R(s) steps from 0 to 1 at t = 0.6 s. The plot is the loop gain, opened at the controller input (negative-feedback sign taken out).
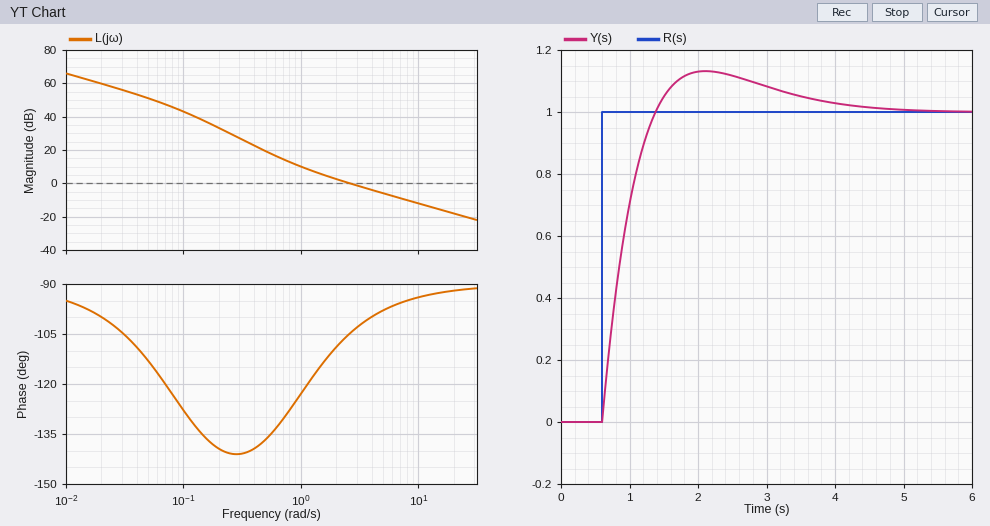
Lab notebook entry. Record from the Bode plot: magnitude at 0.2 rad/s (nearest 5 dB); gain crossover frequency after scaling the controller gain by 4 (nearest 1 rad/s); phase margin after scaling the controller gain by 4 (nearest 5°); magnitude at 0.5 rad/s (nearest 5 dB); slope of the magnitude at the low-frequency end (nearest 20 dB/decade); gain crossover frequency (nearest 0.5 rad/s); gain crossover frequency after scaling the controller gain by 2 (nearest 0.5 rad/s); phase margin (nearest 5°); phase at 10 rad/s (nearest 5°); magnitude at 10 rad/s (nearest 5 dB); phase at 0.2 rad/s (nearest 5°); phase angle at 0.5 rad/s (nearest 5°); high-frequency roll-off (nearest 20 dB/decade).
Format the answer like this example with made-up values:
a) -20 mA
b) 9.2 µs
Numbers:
a) 35 dB
b) 10 rad/s
c) 85°
d) 20 dB
e) -20 dB/decade
f) 2.5 rad/s
g) 5.0 rad/s
h) 75°
i) -95°
j) -10 dB
k) -140°
l) -135°
m) -20 dB/decade
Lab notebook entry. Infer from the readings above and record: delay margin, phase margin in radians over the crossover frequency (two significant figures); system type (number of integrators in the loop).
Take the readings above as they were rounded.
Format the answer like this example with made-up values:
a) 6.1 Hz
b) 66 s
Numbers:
a) 0.52 s
b) 1
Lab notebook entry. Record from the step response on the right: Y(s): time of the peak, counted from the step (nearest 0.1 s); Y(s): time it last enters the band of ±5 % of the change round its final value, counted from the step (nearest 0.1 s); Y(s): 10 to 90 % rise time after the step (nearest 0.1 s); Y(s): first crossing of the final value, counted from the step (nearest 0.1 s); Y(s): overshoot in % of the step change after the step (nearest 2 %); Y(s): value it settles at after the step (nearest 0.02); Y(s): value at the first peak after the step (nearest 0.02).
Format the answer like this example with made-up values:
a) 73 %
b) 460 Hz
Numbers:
a) 1.5 s
b) 2.9 s
c) 0.6 s
d) 0.8 s
e) 14 %
f) 1.00
g) 1.14
